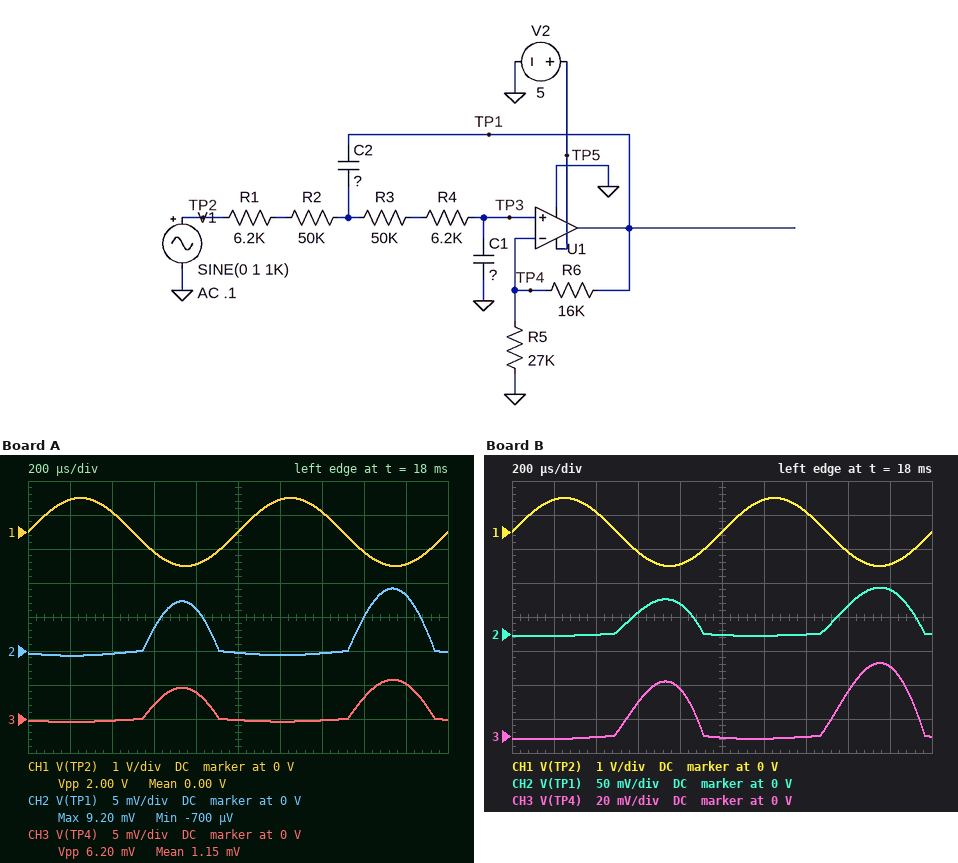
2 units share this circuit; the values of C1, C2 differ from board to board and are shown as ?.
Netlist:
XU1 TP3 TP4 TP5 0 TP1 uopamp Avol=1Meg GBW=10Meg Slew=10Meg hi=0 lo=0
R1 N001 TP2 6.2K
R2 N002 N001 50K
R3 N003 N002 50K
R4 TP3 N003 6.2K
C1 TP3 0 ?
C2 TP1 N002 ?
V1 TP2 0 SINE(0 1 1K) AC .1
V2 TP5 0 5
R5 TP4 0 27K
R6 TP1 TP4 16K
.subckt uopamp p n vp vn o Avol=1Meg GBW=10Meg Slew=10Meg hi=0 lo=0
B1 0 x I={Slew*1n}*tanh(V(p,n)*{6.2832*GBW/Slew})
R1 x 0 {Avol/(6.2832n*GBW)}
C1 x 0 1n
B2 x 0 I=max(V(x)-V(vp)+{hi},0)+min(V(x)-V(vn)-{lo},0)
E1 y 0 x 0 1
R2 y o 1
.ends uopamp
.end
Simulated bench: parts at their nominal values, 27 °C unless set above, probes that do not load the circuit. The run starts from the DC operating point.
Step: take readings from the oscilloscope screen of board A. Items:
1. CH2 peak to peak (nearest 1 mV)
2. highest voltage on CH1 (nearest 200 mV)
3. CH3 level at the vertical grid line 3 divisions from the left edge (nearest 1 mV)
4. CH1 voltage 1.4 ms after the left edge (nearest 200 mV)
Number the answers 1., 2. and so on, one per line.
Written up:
1. 10 mV
2. 1.0 V
3. 2 mV
4. 600 mV
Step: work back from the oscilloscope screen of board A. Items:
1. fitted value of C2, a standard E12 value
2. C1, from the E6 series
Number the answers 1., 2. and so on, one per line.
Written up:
1. 68 nF
2. 15 nF
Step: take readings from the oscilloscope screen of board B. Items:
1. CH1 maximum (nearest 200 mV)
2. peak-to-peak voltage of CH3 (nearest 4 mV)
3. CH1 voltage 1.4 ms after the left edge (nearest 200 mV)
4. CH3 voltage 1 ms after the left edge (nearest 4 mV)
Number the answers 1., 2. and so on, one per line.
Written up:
1. 1.0 V
2. 44 mV
3. 600 mV
4. 0 V
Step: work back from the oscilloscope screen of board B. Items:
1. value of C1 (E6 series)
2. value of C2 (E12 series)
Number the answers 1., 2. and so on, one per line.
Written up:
1. 3.3 nF
2. 56 nF
